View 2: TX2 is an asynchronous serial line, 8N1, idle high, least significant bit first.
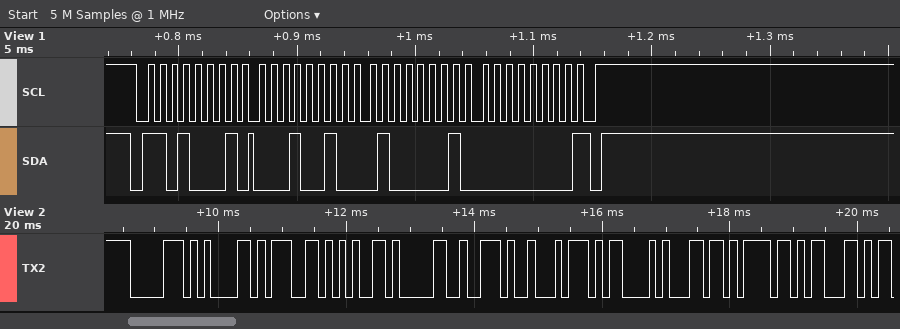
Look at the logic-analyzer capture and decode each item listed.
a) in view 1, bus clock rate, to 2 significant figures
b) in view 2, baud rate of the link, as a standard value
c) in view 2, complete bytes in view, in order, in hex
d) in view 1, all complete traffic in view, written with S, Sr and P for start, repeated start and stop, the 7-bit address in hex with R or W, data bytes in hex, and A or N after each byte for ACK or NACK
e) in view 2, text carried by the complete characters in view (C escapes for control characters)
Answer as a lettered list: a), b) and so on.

a) 100 kHz
b) 9600 baud
c) 70 61 67 65 30 2E 74 43 6C 6F 63
d) S 68R A 12 A 41 A 00 N P
e) "page0.tCloc"
